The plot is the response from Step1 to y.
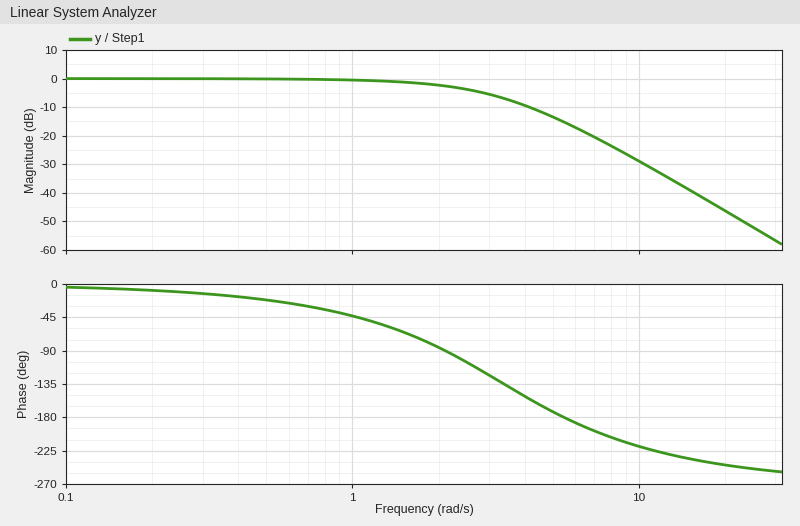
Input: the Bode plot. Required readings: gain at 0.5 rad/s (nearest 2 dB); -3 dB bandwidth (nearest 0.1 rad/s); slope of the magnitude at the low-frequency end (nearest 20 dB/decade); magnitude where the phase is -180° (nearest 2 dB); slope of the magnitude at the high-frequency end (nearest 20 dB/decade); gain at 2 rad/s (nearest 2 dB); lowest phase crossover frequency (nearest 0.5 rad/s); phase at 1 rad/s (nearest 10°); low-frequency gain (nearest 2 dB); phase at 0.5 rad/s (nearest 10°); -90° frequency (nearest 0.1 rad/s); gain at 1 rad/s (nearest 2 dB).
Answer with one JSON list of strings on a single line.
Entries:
["0 dB", "2.3 rad/s", "0 dB/decade", "-16 dB", "-60 dB/decade", "-2 dB", "5.5 rad/s", "-40°", "0 dB", "-20°", "2.1 rad/s", "0 dB"]
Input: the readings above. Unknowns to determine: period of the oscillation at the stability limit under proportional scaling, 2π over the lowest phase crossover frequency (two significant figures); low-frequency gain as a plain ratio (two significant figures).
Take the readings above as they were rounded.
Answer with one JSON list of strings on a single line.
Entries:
["1.1 s", "1.0"]
